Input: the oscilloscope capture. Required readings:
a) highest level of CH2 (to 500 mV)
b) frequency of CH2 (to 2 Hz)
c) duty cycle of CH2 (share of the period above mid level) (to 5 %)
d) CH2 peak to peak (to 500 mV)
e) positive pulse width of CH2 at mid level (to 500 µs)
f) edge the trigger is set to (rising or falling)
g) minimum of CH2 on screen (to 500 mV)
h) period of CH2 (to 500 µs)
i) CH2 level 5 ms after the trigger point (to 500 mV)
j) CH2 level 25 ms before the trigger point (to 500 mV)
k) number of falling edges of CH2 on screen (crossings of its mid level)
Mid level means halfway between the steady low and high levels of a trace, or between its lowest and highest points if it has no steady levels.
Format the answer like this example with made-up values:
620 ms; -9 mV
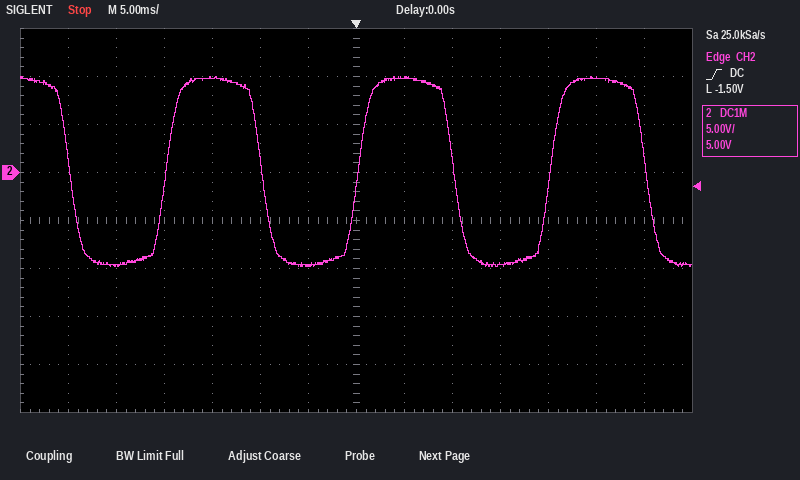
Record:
10.0 V; 50 Hz; 50 %; 20.0 V; 10.0 ms; rising; -10.0 V; 20.0 ms; 10.0 V; -9.5 V; 4
